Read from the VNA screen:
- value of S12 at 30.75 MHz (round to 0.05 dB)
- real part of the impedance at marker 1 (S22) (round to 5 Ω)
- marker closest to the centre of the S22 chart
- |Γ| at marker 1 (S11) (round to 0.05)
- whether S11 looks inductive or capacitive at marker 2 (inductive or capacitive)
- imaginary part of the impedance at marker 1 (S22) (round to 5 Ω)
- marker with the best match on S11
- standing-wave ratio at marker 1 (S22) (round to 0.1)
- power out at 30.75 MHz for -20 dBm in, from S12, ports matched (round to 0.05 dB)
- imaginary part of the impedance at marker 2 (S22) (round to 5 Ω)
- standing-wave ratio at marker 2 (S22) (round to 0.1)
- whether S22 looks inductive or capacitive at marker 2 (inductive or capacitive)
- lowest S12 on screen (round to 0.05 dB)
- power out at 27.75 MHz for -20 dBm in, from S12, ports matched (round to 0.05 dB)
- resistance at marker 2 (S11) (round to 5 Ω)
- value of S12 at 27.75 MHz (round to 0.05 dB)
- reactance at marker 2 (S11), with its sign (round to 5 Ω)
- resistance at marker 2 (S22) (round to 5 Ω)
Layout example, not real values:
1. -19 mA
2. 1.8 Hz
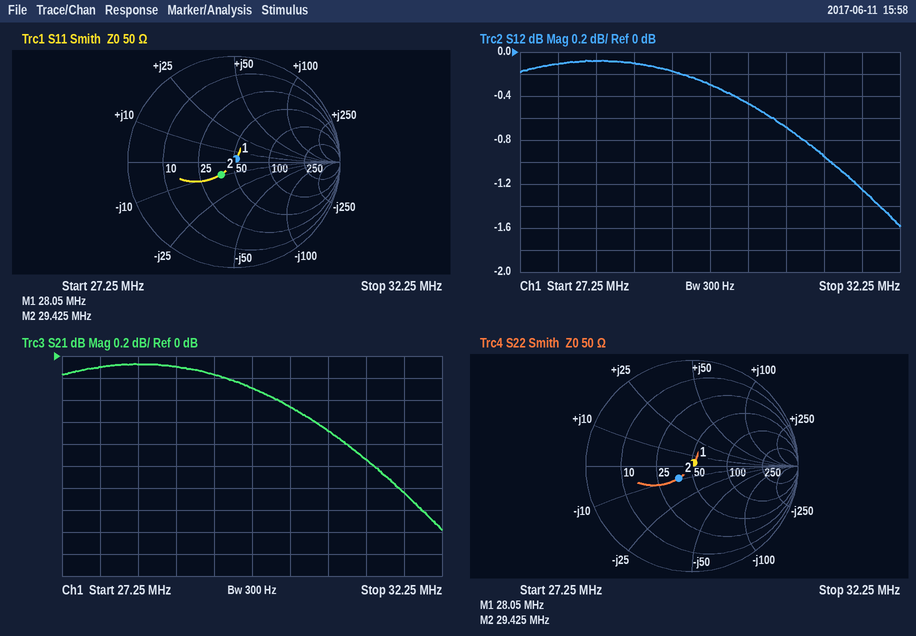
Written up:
1. -0.70 dB
2. 50 Ω
3. marker 1
4. 0.05
5. capacitive
6. +5 Ω
7. marker 1
8. 1.1
9. -20.70 dBm
10. -10 Ω
11. 1.4
12. capacitive
13. -1.60 dB
14. -20.10 dBm
15. 40 Ω
16. -0.10 dB
17. -10 Ω
18. 40 Ω
